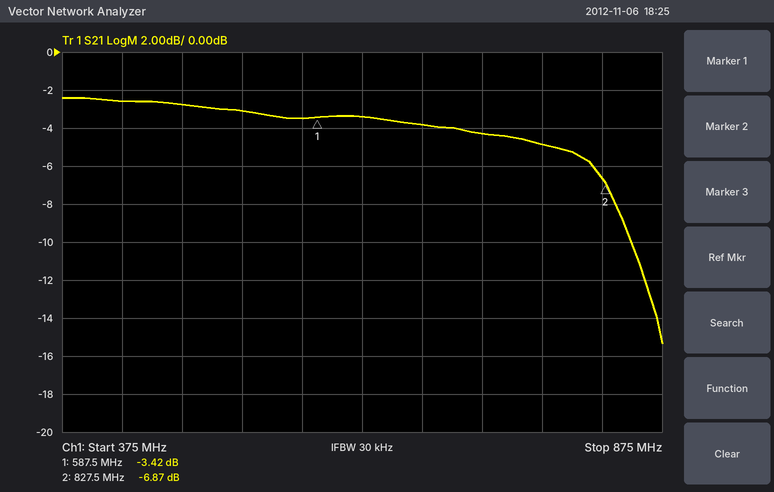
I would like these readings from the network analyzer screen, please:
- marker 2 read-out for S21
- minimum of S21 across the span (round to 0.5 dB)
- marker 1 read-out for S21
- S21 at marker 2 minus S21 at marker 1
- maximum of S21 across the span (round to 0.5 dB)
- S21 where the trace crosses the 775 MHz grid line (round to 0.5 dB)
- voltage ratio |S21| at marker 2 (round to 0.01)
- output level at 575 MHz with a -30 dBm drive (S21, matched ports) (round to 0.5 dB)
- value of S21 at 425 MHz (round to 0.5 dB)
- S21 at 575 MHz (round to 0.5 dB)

-6.87 dB
-15.5 dB
-3.42 dB
-3.45 dB
-2.5 dB
-5.0 dB
0.45
-33.5 dBm
-2.5 dB
-3.5 dB
